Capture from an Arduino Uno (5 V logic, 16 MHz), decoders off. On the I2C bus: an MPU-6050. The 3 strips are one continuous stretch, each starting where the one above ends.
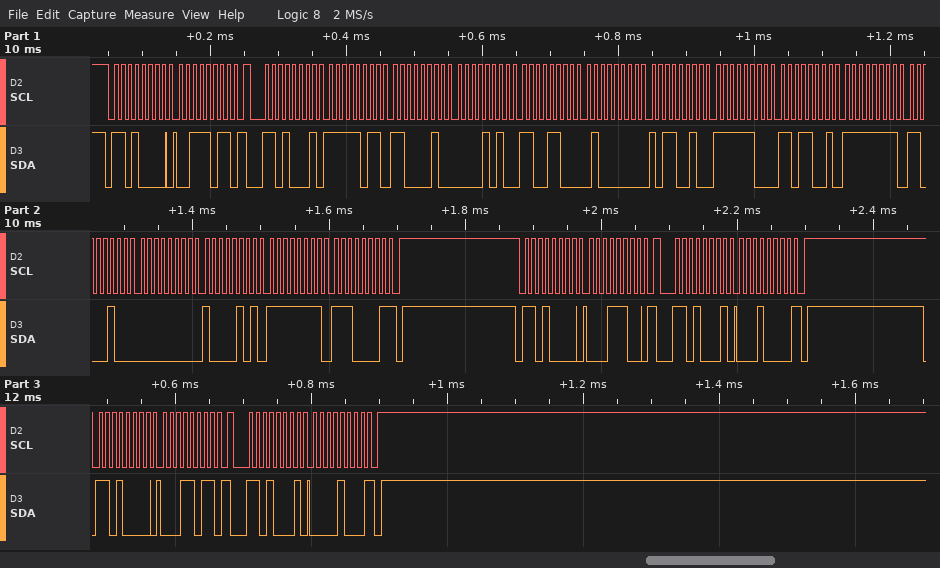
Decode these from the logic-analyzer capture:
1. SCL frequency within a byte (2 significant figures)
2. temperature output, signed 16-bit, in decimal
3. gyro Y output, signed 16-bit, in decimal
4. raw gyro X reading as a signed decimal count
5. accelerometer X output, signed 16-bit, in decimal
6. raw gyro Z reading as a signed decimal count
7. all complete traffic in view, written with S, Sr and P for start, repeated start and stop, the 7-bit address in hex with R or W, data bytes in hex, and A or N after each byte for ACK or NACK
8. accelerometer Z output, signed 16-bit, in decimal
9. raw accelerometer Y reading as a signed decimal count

100 kHz
-807
133
-60
-1086
-31
S 68W A 3B A Sr 68R A FB A C2 A 0A A CC A 40 A B2 A FC A D9 A FF A C4 A 00 A 85 A FF A E1 N P S 68W A 1C A Sr 68R A 10 N P S 68W A 1B A Sr 68R A 08 N P
16562
2764
